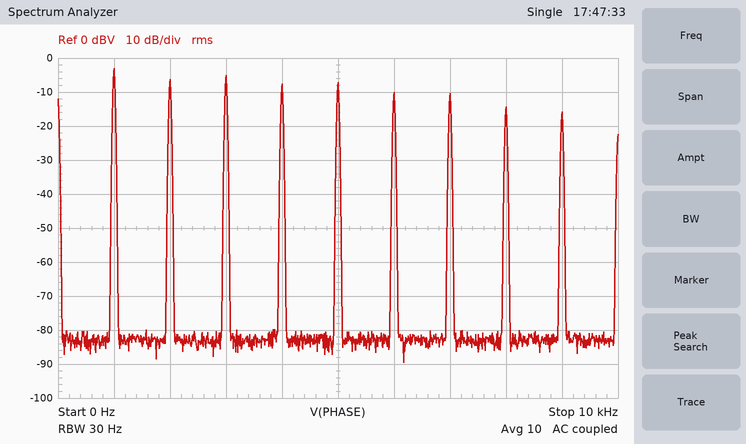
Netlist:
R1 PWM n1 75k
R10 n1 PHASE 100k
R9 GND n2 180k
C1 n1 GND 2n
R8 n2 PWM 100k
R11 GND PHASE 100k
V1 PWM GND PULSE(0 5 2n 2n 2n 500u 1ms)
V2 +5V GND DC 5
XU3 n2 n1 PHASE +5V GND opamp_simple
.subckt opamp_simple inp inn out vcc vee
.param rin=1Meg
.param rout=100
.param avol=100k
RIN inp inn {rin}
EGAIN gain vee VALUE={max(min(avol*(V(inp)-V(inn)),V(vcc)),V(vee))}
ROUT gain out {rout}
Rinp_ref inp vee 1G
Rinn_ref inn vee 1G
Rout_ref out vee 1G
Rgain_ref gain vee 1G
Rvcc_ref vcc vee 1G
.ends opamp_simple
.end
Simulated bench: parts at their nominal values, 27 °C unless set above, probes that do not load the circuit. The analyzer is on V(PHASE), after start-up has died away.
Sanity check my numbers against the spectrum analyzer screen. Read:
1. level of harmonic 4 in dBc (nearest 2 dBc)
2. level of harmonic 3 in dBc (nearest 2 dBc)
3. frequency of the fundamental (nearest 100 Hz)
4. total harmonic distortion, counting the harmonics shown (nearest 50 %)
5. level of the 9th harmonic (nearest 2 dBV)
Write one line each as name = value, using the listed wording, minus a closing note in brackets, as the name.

level of harmonic 4 in dBc = -4 dBc
level of harmonic 3 in dBc = -2 dBc
frequency of the fundamental = 1.0 kHz
total harmonic distortion, counting the harmonics shown = 150 %
level of the 9th harmonic = -16 dBV
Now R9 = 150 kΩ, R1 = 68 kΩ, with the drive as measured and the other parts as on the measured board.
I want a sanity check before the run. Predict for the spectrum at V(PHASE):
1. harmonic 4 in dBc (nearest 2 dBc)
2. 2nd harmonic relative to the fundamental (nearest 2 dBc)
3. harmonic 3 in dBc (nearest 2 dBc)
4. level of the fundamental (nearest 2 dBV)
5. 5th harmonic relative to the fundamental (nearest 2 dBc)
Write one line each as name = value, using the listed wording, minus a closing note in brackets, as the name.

harmonic 4 in dBc = -2 dBc
2nd harmonic relative to the fundamental = 0 dBc
harmonic 3 in dBc = 0 dBc
level of the fundamental = -6 dBV
5th harmonic relative to the fundamental = -2 dBc
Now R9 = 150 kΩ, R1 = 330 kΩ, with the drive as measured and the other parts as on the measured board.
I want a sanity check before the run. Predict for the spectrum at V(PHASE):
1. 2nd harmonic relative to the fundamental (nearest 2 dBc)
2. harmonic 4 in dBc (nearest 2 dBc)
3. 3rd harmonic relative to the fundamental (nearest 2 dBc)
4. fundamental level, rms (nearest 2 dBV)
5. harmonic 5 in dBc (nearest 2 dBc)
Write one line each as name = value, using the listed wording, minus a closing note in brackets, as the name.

2nd harmonic relative to the fundamental = -10 dBc
harmonic 4 in dBc = -14 dBc
3rd harmonic relative to the fundamental = -6 dBc
fundamental level, rms = 2 dBV
harmonic 5 in dBc = -10 dBc
